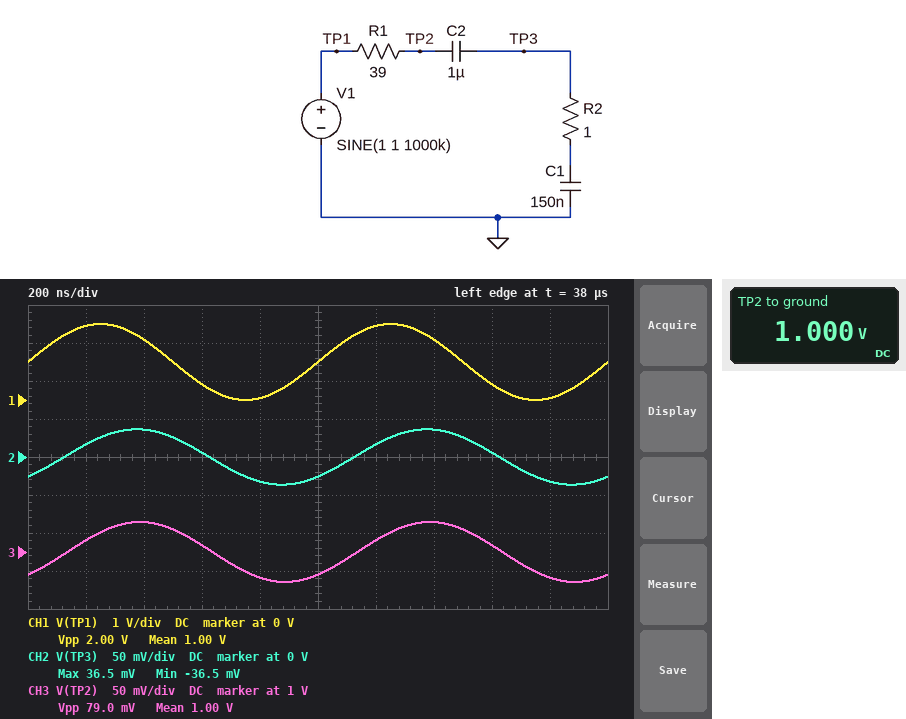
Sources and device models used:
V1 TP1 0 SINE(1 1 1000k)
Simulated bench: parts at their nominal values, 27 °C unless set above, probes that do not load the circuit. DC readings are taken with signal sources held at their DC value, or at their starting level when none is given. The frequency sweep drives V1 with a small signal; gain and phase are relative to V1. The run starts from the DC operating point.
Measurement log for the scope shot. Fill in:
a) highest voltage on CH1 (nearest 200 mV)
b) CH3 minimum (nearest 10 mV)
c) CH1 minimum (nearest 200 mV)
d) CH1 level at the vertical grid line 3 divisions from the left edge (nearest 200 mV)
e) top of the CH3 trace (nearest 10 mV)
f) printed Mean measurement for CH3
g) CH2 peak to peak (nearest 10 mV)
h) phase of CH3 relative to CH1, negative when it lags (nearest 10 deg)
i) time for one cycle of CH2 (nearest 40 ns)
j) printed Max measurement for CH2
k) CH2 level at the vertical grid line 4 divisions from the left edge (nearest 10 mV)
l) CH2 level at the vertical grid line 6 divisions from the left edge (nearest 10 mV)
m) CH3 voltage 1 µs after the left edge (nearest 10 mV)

2.0 V
960 mV
0 V
400 mV
1.04 V
1.00 V
70 mV
-50 deg
1.00 µs
36.5 mV
-30 mV
20 mV
970 mV
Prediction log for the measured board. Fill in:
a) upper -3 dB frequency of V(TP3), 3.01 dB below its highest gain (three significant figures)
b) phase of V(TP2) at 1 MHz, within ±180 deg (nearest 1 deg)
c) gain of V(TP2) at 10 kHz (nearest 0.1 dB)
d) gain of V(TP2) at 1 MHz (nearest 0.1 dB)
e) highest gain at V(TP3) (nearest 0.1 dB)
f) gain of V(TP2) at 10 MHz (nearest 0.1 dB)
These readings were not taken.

30.5 kHz
-49 deg
-0.4 dB
-28.1 dB
-1.2 dB
-32.0 dB
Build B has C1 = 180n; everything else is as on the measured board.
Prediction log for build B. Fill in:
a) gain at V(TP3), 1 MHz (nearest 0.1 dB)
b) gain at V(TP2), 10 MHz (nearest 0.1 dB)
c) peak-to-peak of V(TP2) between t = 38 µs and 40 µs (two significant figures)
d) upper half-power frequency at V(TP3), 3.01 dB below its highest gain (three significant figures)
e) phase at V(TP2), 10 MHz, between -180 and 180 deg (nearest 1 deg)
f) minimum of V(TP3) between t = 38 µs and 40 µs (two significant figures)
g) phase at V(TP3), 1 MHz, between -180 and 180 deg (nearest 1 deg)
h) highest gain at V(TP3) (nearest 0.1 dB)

-29.5 dB
-32.0 dB
72 mV
26.1 kHz
-6 deg
-33 mV
-40 deg
-1.4 dB
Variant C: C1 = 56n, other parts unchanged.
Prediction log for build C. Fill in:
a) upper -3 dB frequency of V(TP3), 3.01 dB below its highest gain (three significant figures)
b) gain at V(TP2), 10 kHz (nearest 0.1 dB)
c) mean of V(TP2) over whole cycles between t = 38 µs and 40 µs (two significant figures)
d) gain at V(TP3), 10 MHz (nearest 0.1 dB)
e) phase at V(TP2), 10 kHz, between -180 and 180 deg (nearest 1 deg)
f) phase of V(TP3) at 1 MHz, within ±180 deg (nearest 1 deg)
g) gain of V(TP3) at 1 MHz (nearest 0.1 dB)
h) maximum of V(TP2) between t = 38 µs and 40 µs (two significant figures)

75.1 kHz
-0.1 dB
1.0 V
-31.7 dB
-7 deg
-66 deg
-22.5 dB
1.1 V
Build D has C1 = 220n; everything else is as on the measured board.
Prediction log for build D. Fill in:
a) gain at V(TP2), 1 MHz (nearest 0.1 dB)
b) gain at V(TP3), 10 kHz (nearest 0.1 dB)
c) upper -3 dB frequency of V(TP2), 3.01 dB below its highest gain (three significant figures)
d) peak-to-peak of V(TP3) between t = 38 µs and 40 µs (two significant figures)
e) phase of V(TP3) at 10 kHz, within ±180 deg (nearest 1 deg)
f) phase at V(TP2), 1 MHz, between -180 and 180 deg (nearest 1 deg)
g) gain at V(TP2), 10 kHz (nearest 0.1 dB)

-29.5 dB
-2.5 dB
22.1 kHz
62 mV
-24 deg
-40 deg
-0.8 dB
